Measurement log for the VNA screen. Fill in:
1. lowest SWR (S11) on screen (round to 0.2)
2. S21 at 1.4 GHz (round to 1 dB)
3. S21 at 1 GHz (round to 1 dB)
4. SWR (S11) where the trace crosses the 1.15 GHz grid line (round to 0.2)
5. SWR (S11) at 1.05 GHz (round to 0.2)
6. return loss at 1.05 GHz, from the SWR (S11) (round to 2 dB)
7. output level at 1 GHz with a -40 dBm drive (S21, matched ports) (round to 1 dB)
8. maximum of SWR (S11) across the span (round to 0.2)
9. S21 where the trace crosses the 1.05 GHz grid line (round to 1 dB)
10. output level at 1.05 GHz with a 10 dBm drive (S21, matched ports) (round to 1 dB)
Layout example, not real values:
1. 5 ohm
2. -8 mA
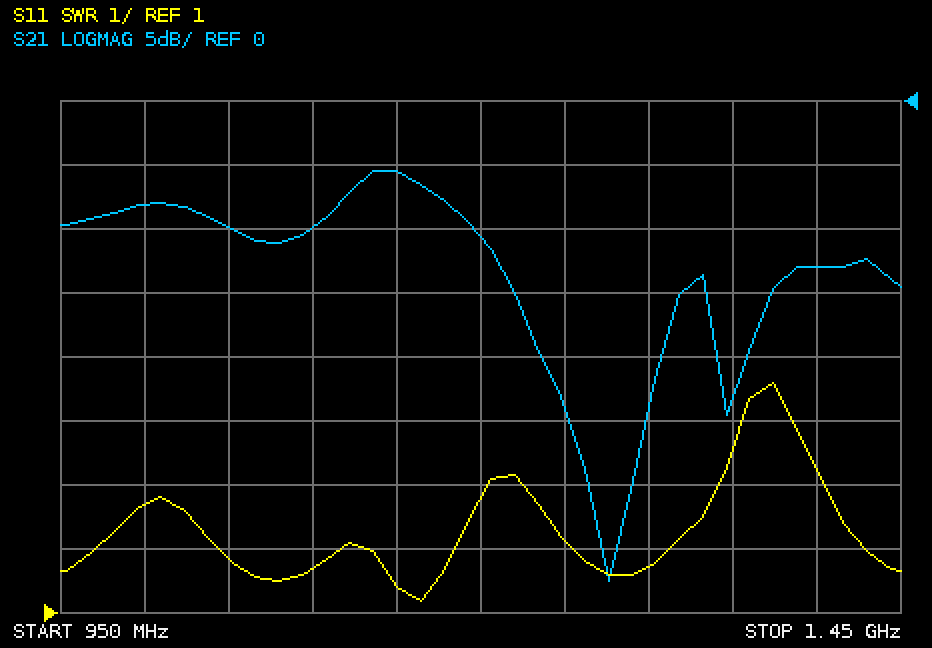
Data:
1. 1.2
2. -13 dB
3. -8 dB
4. 1.4
5. 1.8
6. 10 dB
7. -48 dBm
8. 4.6
9. -10 dB
10. 0 dBm
